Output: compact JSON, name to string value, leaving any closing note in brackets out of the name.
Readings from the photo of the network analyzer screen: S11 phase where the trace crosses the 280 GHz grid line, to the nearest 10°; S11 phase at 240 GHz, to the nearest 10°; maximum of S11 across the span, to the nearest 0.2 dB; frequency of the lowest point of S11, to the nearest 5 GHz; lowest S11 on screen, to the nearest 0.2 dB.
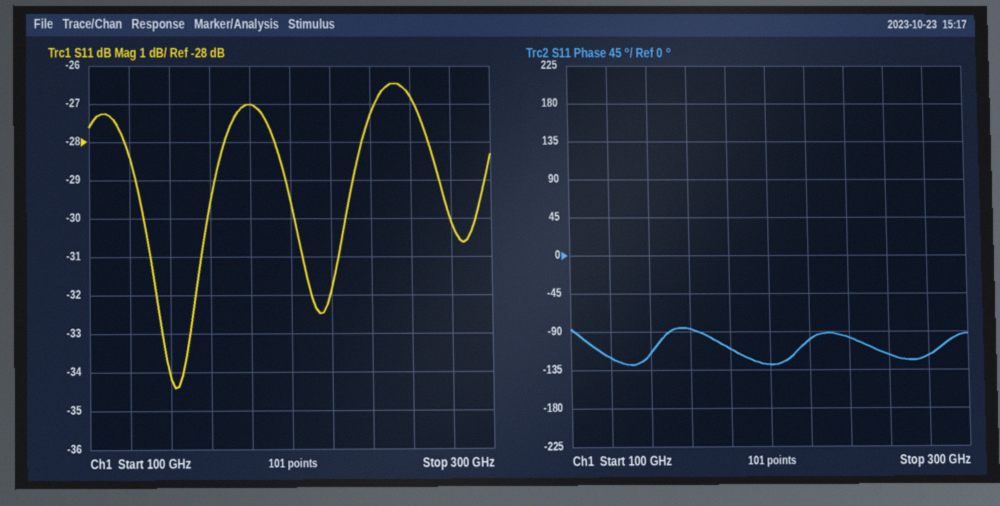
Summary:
{"S11 phase where the trace crosses the 280 GHz grid line, to the nearest 10°": "-120°", "S11 phase at 240 GHz, to the nearest 10°": "-100°", "maximum of S11 across the span, to the nearest 0.2 dB": "-26.4 dB", "frequency of the lowest point of S11, to the nearest 5 GHz": "140 GHz", "lowest S11 on screen, to the nearest 0.2 dB": "-34.4 dB"}
